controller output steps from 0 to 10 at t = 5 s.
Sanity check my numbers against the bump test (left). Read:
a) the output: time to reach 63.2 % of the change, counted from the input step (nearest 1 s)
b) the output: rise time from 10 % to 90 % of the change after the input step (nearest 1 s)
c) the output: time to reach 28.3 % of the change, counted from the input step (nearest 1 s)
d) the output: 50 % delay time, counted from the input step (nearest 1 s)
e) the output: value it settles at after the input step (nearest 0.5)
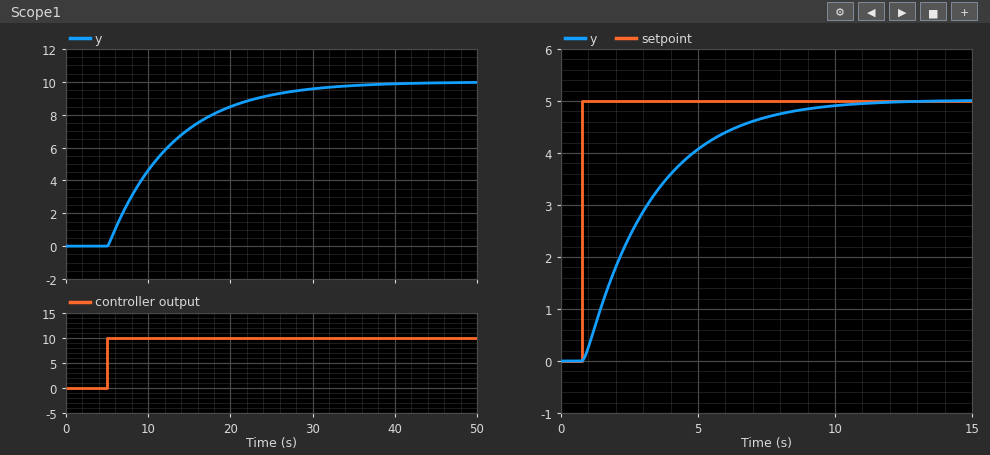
8 s
17 s
3 s
6 s
10.0
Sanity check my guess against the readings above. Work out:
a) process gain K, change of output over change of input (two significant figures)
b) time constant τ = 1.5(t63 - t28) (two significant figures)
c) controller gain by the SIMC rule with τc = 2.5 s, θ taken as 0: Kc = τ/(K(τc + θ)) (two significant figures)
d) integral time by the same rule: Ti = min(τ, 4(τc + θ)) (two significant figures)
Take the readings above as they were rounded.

1.0
7.5 s
3.0
7.5 s
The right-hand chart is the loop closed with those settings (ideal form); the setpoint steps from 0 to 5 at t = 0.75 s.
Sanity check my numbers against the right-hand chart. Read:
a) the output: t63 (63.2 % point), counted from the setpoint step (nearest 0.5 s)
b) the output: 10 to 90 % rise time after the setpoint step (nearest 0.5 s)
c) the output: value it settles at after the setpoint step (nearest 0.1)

2.5 s
5.5 s
5.0
